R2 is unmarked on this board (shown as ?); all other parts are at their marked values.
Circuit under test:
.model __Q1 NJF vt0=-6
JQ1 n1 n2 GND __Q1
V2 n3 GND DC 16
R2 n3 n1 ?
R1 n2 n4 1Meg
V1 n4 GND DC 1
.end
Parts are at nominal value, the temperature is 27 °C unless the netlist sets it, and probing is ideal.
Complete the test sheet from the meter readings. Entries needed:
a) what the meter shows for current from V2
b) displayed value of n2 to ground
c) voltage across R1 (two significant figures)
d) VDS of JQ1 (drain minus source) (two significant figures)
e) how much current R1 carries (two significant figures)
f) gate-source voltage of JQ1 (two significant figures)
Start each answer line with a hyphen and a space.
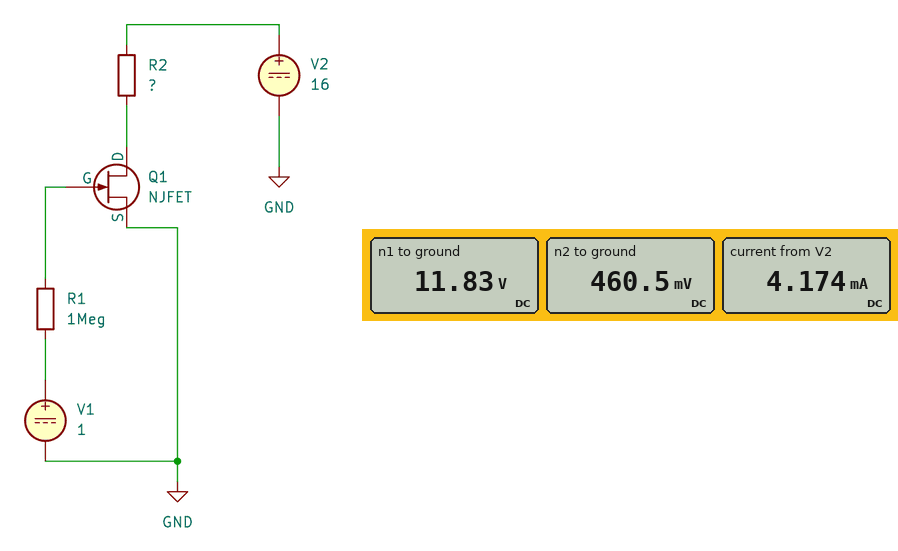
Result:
- 4.174 mA
- 460.5 mV
- 540 mV
- 12 V
- 540 nA
- 460 mV
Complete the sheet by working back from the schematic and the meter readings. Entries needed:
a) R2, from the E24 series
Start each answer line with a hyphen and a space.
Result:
- 1 kΩ
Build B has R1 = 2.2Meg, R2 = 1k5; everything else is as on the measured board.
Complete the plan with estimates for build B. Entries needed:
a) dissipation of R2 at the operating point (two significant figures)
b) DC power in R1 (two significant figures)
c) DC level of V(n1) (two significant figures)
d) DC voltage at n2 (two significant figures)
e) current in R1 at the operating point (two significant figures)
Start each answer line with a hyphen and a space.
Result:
- 26 mW
- 140 nW
- 9.8 V
- 440 mV
- 250 nA
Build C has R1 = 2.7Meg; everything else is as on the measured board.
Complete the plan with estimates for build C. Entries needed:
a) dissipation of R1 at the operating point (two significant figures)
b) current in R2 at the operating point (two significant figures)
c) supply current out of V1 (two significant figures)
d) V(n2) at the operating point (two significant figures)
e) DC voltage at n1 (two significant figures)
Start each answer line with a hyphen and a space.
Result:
- 120 nW
- 4.1 mA
- 210 nA
- 440 mV
- 12 V
